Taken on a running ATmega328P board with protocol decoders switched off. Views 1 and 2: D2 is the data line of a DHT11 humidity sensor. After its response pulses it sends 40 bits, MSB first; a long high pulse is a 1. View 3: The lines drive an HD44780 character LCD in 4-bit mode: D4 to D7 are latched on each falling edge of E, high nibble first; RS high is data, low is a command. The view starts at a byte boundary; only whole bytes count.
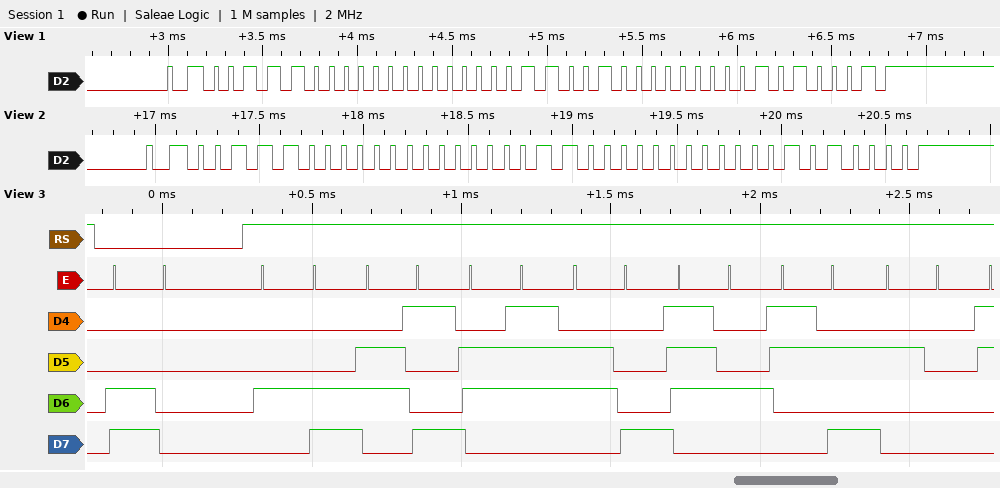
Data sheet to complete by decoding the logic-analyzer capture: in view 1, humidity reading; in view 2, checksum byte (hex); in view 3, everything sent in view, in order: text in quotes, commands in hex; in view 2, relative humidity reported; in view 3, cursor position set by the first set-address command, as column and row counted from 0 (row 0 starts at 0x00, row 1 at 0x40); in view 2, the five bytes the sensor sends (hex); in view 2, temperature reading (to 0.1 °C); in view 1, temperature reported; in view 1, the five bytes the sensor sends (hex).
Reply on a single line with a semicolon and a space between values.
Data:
56 %; 0x50; 0xC0 "Light: "; 56 %; column 0, row 1; 38 00 18 00 50; 24.0 °C; 25.0 °C; 38 00 19 00 51
